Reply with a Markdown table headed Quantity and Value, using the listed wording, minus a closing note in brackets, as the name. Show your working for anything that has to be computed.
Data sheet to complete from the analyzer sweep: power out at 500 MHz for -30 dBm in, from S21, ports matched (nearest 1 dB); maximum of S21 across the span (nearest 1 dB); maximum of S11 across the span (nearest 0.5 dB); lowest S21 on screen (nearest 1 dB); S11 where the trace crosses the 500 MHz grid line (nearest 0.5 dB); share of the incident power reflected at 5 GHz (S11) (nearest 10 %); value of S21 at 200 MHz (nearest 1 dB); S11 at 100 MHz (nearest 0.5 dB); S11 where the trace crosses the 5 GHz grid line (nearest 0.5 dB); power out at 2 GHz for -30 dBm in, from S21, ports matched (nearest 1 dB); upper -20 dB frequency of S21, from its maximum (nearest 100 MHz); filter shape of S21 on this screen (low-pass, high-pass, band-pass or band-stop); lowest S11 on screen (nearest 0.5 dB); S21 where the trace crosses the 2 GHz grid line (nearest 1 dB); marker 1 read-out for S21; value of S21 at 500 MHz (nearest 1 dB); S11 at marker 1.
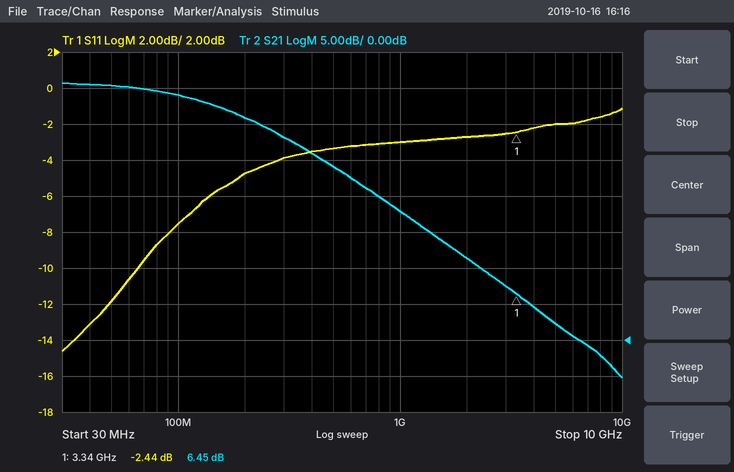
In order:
| Quantity | Value |
|---|---|
| power out at 500 MHz for -30 dBm in, from S21, ports matched | -30 dBm + (24 dB) = -6 dBm |
| maximum of S21 across the span | 36 dB |
| maximum of S11 across the span | -1.0 dB |
| lowest S21 on screen | -5 dB |
| S11 where the trace crosses the 500 MHz grid line | -3.5 dB |
| share of the incident power reflected at 5 GHz (S11) | 10^(-2/10) ≈ 63.1 %, so 60 % to the nearest 10 % |
| value of S21 at 200 MHz | 31 dB |
| S11 at 100 MHz | -7.5 dB |
| S11 where the trace crosses the 5 GHz grid line | -2.0 dB |
| power out at 2 GHz for -30 dBm in, from S21, ports matched | -30 dBm + (11 dB) = -19 dBm |
| upper -20 dB frequency of S21, from its maximum | 1.3 GHz |
| filter shape of S21 on this screen | low-pass |
| lowest S11 on screen | -14.5 dB |
| S21 where the trace crosses the 2 GHz grid line | 11 dB |
| marker 1 read-out for S21 | 6.45 dB |
| value of S21 at 500 MHz | 24 dB |
| S11 at marker 1 | -2.44 dB |
